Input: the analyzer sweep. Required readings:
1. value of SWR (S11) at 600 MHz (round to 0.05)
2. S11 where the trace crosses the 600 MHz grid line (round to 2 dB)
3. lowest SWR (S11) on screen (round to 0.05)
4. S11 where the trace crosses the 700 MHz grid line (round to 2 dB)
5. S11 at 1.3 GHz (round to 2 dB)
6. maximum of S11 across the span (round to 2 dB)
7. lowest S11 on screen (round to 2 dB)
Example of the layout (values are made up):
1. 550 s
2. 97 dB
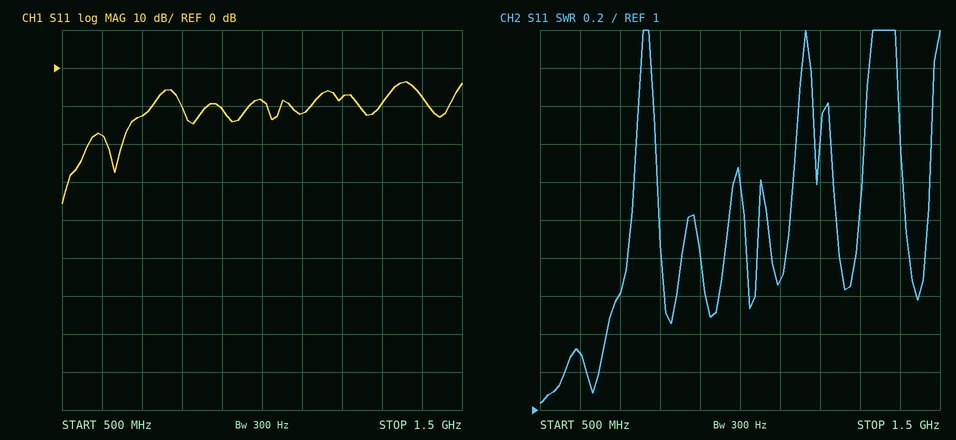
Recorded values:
1. 1.30
2. -18 dB
3. 1.05
4. -12 dB
5. -10 dB
6. -4 dB
7. -36 dB
